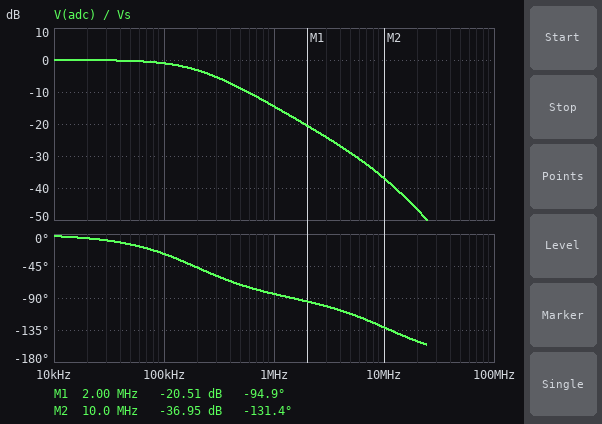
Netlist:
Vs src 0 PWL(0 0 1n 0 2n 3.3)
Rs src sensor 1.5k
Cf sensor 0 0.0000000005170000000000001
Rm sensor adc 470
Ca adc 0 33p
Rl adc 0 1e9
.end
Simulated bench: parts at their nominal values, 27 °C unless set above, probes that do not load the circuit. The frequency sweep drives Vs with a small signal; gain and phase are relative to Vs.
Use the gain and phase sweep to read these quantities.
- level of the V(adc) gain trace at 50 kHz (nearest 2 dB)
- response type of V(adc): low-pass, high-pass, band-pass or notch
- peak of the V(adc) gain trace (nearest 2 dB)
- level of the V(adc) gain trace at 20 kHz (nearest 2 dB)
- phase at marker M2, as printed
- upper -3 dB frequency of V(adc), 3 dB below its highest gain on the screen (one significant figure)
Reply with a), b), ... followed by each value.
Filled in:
a) 0 dB
b) low-pass
c) 0 dB
d) 0 dB
e) -131.4 deg
f) 200 kHz
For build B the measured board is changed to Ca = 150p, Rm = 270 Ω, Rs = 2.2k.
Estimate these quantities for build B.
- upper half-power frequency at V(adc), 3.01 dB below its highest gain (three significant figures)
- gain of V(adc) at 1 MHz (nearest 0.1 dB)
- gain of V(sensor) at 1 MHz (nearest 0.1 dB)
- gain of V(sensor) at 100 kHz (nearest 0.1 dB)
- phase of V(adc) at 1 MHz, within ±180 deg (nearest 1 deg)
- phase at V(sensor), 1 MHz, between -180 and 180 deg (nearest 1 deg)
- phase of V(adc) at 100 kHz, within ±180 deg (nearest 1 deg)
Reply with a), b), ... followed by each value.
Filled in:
a) 108 kHz
b) -19.6 dB
c) -19.3 dB
d) -2.7 dB
e) -95 deg
f) -81 deg
g) -44 deg
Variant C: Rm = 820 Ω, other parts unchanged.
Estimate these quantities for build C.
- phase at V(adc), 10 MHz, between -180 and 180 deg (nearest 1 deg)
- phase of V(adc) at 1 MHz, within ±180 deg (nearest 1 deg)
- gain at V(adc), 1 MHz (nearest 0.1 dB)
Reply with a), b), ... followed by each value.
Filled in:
a) -147 deg
b) -88 deg
c) -14.6 dB
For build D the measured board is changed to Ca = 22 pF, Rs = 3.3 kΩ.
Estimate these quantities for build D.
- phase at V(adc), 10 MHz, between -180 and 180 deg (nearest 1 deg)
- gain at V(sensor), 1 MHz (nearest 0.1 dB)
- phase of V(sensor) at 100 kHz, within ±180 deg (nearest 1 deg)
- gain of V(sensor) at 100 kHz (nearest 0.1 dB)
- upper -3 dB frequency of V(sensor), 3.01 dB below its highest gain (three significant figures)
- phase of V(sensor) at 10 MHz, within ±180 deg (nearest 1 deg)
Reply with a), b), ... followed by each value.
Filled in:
a) -121 deg
b) -21.0 dB
c) -48 deg
d) -3.5 dB
e) 89.5 kHz
f) -88 deg
